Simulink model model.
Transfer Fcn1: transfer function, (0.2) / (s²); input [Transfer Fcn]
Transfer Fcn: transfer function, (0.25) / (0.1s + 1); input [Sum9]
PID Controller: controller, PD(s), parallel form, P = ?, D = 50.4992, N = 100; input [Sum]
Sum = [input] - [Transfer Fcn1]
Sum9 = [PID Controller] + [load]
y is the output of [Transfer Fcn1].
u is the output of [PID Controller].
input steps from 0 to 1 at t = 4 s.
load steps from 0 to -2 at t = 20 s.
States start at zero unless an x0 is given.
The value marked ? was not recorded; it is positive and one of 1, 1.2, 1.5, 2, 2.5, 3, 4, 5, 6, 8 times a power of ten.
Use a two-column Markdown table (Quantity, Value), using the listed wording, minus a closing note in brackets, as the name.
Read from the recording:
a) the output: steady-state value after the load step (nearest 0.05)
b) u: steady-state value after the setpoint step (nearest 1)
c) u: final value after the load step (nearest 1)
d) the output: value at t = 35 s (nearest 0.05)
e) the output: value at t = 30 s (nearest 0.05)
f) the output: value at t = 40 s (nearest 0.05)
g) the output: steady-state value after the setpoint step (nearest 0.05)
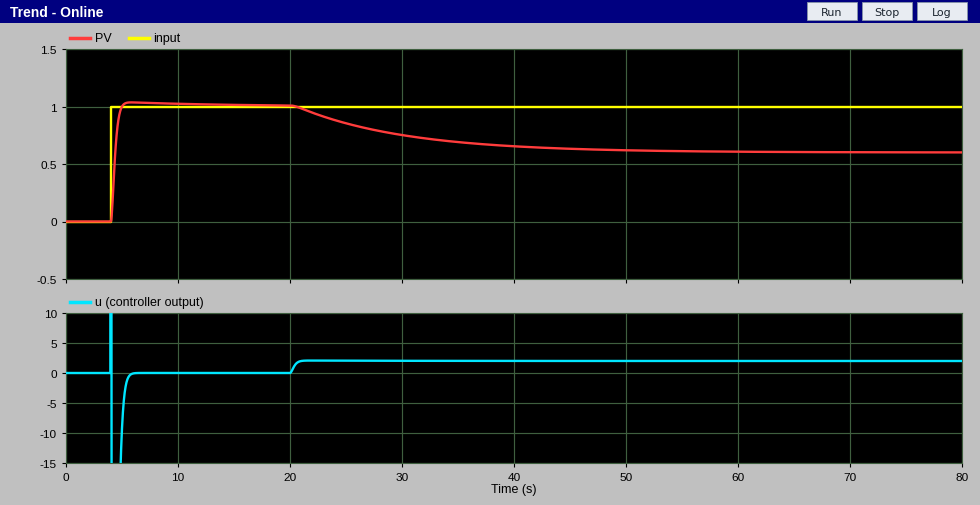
| Quantity | Value |
|---|---|
| the output: steady-state value after the load step | 0.60 |
| u: steady-state value after the setpoint step | 0 |
| u: final value after the load step | 2 |
| the output: value at t = 35 s | 0.70 |
| the output: value at t = 30 s | 0.75 |
| the output: value at t = 40 s | 0.65 |
| the output: steady-state value after the setpoint step | 1.00 |
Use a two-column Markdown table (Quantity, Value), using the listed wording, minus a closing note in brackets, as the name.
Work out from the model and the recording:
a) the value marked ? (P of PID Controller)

| Quantity | Value |
|---|---|
| the value marked ? | 5 |
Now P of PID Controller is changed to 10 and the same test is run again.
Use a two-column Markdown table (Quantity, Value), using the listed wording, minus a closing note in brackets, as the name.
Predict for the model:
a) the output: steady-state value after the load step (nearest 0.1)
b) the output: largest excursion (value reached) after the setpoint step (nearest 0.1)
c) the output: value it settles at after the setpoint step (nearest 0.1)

| Quantity | Value |
|---|---|
| the output: steady-state value after the load step | 0.8 |
| the output: largest excursion (value reached) after the setpoint step | 1.1 |
| the output: value it settles at after the setpoint step | 1.0 |
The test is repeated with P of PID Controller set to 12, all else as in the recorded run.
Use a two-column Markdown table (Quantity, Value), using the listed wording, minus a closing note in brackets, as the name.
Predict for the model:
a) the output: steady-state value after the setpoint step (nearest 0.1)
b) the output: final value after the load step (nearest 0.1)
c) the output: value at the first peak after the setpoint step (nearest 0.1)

| Quantity | Value |
|---|---|
| the output: steady-state value after the setpoint step | 1.0 |
| the output: final value after the load step | 0.8 |
| the output: value at the first peak after the setpoint step | 1.1 |
